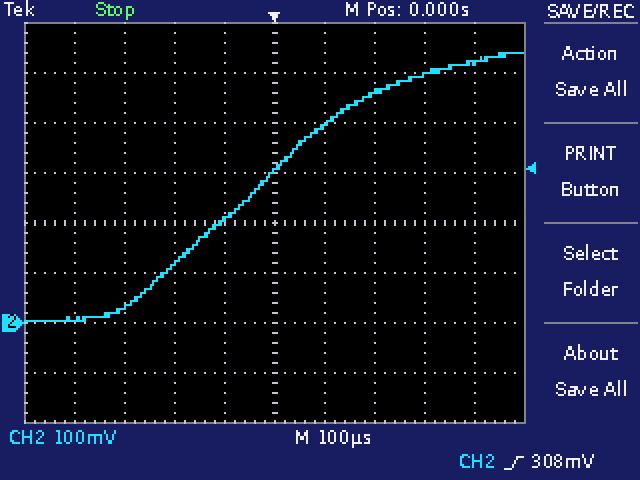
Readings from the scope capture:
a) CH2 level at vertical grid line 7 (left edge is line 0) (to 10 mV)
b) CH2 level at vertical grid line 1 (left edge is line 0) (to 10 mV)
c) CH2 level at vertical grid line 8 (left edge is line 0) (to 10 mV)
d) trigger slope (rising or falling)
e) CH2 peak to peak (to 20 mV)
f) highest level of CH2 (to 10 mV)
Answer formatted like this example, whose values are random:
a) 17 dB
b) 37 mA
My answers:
a) 460 mV
b) 10 mV
c) 500 mV
d) rising
e) 540 mV
f) 540 mV
